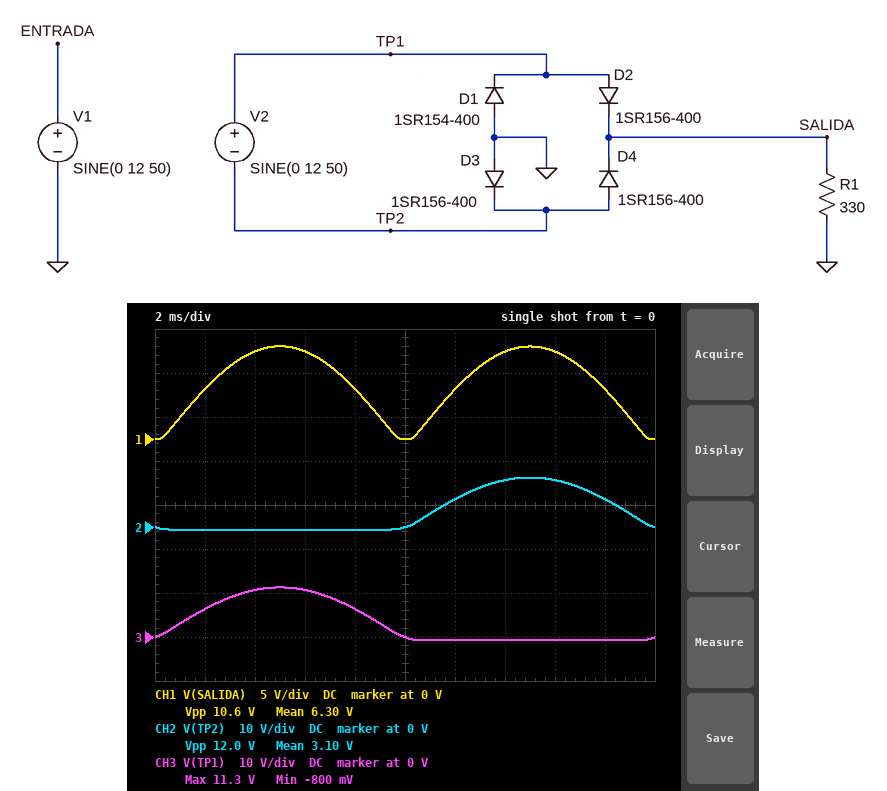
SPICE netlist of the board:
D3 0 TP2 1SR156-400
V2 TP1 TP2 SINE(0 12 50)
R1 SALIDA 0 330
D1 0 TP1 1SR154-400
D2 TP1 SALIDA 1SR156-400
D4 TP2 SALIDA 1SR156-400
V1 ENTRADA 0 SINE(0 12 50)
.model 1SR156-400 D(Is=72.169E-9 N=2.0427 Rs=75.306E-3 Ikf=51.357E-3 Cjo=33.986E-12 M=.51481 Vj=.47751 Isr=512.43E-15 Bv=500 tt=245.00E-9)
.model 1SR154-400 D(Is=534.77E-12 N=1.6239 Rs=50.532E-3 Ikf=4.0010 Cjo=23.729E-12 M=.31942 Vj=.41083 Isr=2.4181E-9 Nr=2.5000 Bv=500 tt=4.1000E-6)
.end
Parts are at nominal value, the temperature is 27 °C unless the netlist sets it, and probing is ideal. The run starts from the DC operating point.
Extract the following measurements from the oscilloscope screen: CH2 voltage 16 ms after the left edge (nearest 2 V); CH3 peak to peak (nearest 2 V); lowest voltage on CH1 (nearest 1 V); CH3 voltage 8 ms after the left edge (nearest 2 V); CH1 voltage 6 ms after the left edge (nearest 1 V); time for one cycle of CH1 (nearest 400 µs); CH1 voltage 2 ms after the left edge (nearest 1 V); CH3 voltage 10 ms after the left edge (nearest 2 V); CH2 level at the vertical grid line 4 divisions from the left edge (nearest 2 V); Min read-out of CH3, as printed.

10 V
12 V
0 V
6 V
10 V
10.0 ms
6 V
0 V
0 V
-800 mV
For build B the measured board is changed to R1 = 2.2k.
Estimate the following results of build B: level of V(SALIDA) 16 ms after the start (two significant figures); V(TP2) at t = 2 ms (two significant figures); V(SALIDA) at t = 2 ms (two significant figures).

10 V
-570 mV
5.9 V
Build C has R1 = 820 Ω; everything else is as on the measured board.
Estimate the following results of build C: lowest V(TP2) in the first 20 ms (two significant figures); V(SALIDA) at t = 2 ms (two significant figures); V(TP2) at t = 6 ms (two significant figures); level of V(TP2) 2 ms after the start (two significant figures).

-670 mV
5.8 V
-660 mV
-630 mV
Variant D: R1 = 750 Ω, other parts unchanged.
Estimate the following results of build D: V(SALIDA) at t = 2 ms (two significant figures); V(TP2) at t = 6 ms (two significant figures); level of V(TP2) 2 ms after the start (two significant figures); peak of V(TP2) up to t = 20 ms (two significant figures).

5.8 V
-670 mV
-630 mV
11 V
